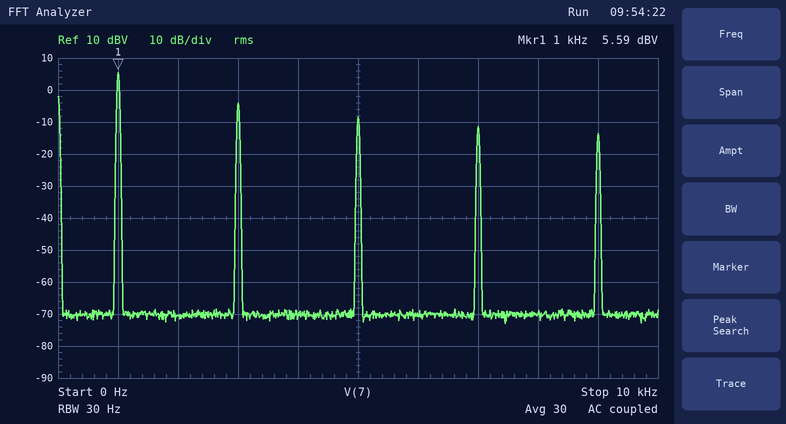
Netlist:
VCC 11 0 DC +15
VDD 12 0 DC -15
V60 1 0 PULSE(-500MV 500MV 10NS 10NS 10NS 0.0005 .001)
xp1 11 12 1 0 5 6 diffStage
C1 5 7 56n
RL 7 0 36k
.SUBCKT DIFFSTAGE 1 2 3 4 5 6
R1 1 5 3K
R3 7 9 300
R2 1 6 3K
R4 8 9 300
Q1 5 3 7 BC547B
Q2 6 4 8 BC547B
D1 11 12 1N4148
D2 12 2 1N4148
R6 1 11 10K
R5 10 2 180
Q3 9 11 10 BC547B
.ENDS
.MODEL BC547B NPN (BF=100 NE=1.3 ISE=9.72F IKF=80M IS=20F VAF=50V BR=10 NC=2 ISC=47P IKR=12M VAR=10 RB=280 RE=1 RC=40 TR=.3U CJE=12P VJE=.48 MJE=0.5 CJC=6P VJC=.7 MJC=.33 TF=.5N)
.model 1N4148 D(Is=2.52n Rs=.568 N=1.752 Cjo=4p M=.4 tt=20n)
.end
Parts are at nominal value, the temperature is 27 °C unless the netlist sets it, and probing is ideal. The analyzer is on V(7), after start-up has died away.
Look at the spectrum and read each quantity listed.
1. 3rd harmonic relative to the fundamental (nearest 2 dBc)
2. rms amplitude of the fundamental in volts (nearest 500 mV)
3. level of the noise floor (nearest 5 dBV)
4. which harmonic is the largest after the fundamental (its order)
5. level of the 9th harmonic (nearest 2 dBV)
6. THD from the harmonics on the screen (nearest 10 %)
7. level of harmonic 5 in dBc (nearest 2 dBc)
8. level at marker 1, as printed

-10 dBc
2.0 V
-70 dBV
3
-14 dBV
40 %
-14 dBc
5.59 dBV
